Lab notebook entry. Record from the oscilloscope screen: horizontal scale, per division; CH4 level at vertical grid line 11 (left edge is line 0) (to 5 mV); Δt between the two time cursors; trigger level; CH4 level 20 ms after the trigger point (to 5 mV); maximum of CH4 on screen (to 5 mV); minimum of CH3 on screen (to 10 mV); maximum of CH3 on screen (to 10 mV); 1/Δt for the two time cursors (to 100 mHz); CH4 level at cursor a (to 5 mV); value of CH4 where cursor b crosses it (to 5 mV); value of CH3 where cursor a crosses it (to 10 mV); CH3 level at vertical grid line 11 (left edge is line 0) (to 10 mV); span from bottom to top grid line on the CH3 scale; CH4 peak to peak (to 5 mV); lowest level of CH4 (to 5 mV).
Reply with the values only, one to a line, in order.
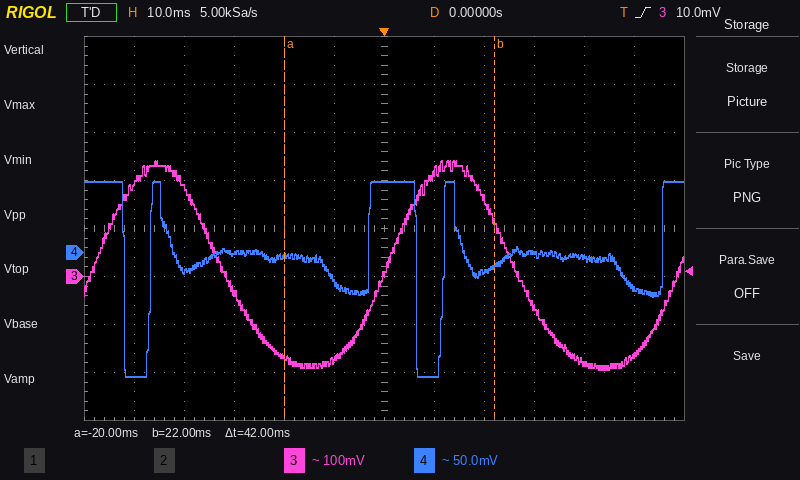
10 ms
-35 mV
42 ms
10.0 mV
-20 mV
75 mV
-190 mV
240 mV
23.8 Hz
-5 mV
-15 mV
-170 mV
-160 mV
800 mV
205 mV
-130 mV
